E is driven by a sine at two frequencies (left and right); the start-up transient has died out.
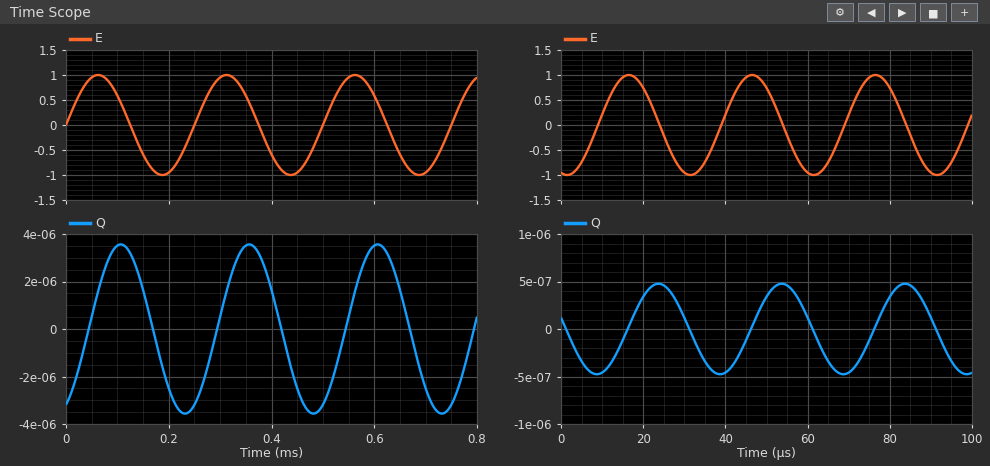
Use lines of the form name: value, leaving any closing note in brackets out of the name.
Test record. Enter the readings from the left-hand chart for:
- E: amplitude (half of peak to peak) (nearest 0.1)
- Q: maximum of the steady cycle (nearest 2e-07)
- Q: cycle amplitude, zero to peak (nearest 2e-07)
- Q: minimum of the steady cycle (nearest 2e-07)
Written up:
E: amplitude (half of peak to peak): 1.0
Q: maximum of the steady cycle: 0.0000036
Q: cycle amplitude, zero to peak: 0.0000036
Q: minimum of the steady cycle: -0.0000036
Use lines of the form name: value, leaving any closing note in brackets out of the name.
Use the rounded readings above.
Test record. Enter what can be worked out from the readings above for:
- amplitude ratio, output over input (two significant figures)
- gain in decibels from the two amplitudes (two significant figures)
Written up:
amplitude ratio, output over input: 0.0000036
gain in decibels from the two amplitudes: -110 dB
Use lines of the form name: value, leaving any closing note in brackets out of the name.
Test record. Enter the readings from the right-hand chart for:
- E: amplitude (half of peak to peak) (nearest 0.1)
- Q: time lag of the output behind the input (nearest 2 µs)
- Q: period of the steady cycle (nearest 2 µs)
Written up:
E: amplitude (half of peak to peak): 1.0
Q: time lag of the output behind the input: 8 µs
Q: period of the steady cycle: 30 µs
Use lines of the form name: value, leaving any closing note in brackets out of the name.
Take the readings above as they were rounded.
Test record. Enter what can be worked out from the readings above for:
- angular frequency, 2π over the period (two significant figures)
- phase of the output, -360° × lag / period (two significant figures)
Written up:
angular frequency, 2π over the period: 0.21 rad/µs
phase of the output, -360° × lag / period: -96°
